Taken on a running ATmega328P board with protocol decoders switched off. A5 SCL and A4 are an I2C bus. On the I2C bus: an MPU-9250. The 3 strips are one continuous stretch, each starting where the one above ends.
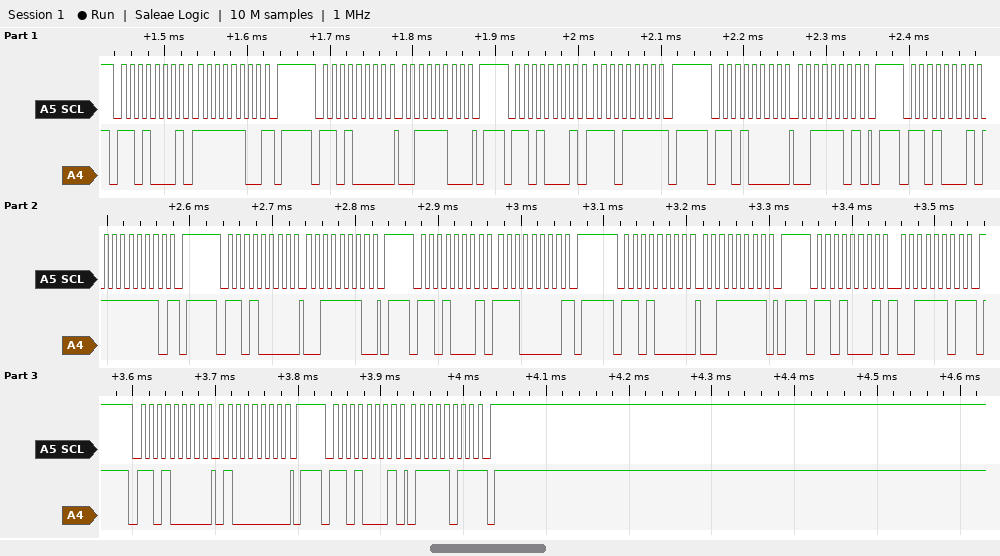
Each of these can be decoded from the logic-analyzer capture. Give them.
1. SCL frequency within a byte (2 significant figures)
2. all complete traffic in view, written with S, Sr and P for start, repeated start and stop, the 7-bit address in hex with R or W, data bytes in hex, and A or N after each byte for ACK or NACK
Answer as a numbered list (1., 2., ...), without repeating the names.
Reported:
1. 100 kHz
2. S 68R A FC N P S 68W A 3C A P S 68R A EF N P S 68W A 3D A P S 68R A FE N P S 68W A 3E A P S 68R A E0 N P S 68W A 3F A P S 68R A 3D N P S 68W A 40 A P S 68R A 7B N P
